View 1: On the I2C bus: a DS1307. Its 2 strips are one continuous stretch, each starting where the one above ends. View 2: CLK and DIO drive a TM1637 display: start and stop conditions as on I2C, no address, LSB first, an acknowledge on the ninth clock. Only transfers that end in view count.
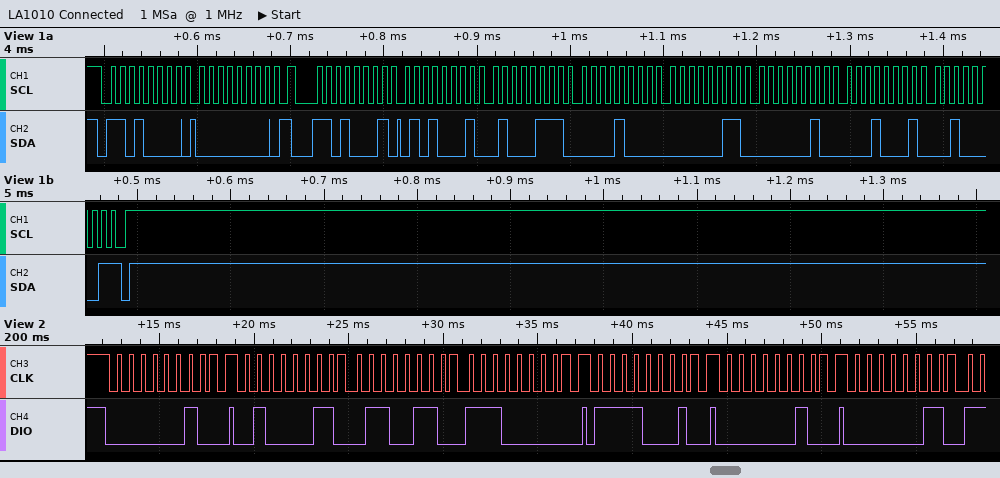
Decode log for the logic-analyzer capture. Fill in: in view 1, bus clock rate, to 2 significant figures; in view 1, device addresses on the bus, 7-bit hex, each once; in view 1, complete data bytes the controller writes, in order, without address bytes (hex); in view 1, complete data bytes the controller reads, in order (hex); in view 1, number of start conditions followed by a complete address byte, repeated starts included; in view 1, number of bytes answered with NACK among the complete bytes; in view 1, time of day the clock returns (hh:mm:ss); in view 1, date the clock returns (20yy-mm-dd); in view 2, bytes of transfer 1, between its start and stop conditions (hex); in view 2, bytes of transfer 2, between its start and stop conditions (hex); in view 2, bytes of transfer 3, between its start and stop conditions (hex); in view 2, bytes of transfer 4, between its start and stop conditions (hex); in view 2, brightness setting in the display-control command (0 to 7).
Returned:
100 kHz
0x68
00
51 47 08 03 02 11 21
2
1
08:47:51
2021-11-02
40
C2 66 07
8F
40
7
